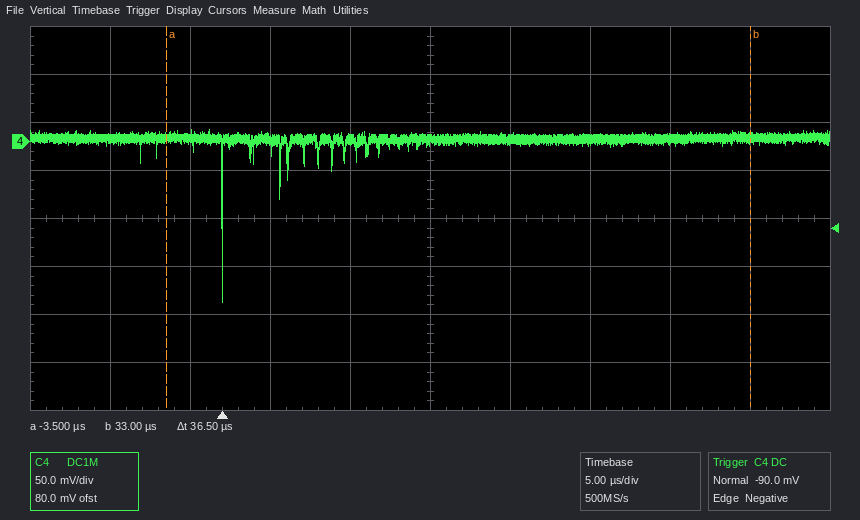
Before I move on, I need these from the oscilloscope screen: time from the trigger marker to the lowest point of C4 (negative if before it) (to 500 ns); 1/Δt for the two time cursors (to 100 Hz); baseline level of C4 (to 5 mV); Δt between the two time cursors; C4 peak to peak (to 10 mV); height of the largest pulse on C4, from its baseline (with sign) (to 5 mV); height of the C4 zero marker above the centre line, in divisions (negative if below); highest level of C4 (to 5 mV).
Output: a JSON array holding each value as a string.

["0.0 µs", "27.4 kHz", "5 mV", "36.5 µs", "180 mV", "-170 mV", "+1.6 div", "15 mV"]
